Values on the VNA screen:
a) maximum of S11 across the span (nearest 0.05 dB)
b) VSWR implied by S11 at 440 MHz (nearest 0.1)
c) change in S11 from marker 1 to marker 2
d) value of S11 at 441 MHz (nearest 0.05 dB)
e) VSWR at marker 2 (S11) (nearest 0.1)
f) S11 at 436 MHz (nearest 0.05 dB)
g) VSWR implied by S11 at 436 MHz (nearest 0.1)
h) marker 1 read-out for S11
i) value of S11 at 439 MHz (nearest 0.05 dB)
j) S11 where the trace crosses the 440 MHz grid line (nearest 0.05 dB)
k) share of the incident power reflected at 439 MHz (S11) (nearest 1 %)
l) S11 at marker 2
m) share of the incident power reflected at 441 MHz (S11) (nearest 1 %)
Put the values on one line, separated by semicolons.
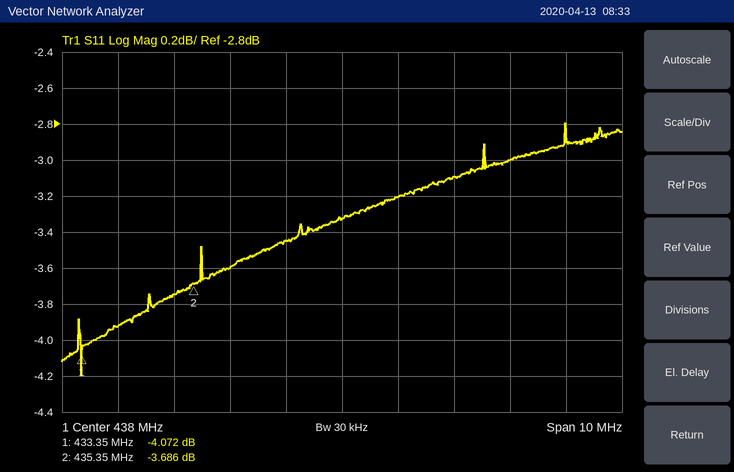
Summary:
-2.80 dB; 5.7; 0.386 dB; -3.00 dB; 4.8; -3.60 dB; 4.9; -4.072 dB; -3.20 dB; -3.10 dB; 48 %; -3.686 dB; 50 %
